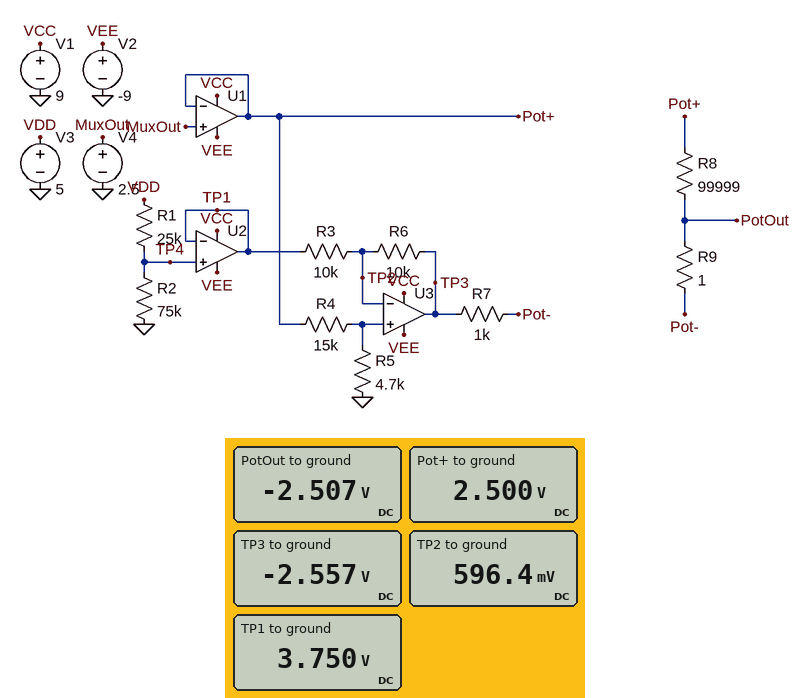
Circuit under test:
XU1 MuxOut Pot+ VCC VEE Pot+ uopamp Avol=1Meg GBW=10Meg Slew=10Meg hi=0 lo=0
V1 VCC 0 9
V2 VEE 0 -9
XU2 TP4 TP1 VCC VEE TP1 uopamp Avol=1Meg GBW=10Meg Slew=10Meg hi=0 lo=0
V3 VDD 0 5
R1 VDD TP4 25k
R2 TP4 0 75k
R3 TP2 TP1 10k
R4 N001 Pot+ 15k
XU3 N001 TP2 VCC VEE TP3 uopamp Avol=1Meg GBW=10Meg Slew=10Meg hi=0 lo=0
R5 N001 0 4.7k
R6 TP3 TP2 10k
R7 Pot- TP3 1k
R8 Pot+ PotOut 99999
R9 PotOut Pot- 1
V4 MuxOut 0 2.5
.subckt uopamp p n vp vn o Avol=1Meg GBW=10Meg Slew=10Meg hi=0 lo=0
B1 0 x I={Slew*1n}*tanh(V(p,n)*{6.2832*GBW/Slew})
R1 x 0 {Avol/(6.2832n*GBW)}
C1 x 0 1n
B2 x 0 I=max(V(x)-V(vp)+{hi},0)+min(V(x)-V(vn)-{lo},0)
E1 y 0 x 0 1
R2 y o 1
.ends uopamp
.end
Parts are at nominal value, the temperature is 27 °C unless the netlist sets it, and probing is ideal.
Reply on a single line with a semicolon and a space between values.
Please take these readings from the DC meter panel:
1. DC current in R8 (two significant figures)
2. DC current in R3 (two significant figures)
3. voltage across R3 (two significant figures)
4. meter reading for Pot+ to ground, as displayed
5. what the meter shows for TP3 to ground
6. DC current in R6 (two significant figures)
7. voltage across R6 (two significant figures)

50 µA; 320 µA; 3.2 V; 2.500 V; -2.557 V; 320 µA; 3.2 V
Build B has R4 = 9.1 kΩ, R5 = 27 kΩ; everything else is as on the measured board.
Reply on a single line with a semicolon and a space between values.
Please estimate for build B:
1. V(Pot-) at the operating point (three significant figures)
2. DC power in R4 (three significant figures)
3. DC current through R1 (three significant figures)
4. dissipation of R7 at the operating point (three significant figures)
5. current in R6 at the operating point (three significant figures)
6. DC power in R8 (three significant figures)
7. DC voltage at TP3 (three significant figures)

14.5 mV; 43.6 µW; 50.0 µA; 618 nW; 188 µA; 61.8 µW; -10.4 mV
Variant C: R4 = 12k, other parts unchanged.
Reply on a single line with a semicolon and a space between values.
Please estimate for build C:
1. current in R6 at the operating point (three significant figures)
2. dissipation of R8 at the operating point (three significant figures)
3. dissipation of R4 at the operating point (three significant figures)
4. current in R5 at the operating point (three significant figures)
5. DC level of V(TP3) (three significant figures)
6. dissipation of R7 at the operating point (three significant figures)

305 µA; 230 µW; 269 µW; 150 µA; -2.34 V; 2.30 µW
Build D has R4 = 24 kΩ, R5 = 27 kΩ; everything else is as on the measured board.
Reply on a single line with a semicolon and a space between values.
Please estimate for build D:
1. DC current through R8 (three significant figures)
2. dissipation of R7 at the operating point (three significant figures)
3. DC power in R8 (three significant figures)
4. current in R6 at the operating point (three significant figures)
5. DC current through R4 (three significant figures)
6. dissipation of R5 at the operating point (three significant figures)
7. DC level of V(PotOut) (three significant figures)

35.7 µA; 1.27 µW; 127 µW; 243 µA; 49.0 µA; 64.9 µW; -1.07 V
